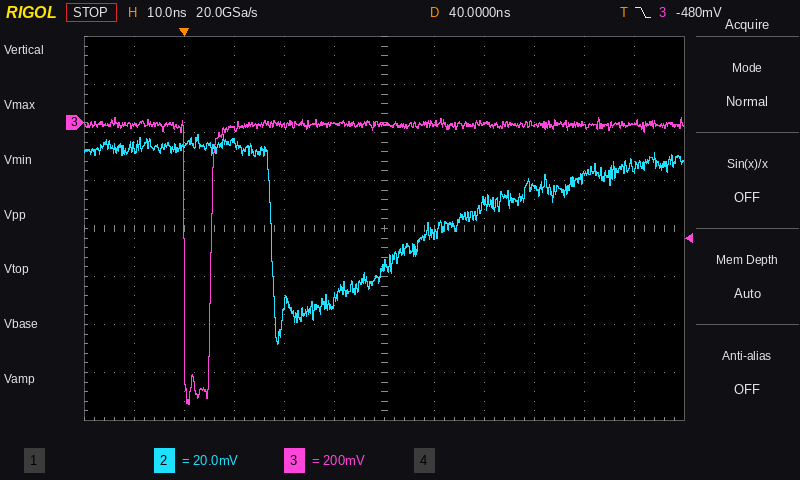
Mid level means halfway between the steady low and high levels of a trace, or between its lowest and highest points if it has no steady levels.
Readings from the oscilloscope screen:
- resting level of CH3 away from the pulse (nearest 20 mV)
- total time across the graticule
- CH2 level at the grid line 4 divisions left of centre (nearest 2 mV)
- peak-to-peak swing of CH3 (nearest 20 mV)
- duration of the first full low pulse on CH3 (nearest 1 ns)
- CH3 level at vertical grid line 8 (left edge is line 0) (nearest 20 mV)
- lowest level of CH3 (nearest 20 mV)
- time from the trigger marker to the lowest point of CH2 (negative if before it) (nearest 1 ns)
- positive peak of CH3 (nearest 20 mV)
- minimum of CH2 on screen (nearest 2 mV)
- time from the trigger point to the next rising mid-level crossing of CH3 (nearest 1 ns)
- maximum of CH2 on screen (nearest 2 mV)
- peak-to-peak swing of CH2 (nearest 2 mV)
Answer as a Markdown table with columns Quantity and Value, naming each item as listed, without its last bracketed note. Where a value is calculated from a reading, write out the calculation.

| Quantity | Value |
|---|---|
| resting level of CH3 away from the pulse | 0 mV |
| total time across the graticule | 120 ns |
| CH2 level at the grid line 4 divisions left of centre | -10 mV |
| peak-to-peak swing of CH3 | 20 mV − (-1.18 V) = 1.20 V |
| duration of the first full low pulse on CH3 | 5 ns |
| CH3 level at vertical grid line 8 (left edge is line 0) | 0 mV |
| lowest level of CH3 | -1.18 V |
| time from the trigger marker to the lowest point of CH2 (negative if before it) | +19 ns |
| positive peak of CH3 | 20 mV |
| minimum of CH2 on screen | -92 mV |
| time from the trigger point to the next rising mid-level crossing of CH3 | 5 ns |
| maximum of CH2 on screen | -4 mV |
| peak-to-peak swing of CH2 | -4 mV − (-92 mV) = 88 mV |
